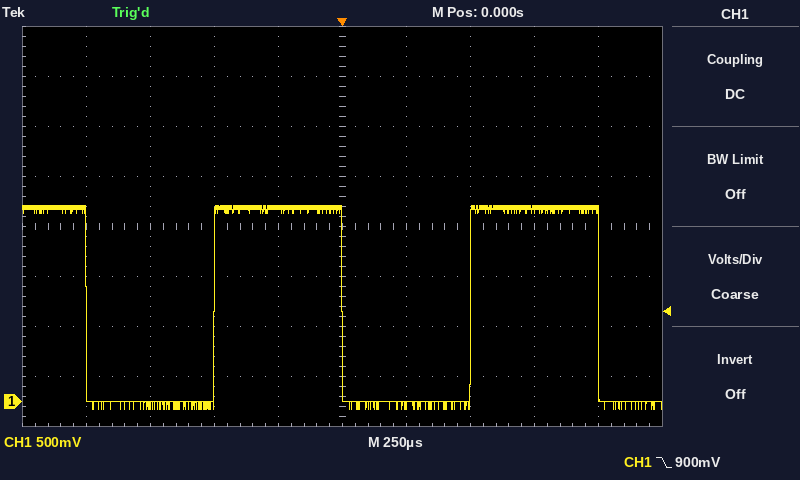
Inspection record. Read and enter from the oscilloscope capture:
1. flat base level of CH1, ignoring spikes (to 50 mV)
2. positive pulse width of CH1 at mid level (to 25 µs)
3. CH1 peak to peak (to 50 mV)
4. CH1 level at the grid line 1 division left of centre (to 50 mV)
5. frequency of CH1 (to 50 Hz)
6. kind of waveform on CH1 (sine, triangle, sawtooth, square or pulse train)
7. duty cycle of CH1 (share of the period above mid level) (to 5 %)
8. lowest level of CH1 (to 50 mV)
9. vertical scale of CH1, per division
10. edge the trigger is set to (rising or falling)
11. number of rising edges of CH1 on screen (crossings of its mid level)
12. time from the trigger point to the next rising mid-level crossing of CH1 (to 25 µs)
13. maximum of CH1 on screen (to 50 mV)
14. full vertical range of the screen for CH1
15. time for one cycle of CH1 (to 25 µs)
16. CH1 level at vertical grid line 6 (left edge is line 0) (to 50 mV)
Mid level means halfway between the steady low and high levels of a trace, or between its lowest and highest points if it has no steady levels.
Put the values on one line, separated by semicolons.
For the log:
0 mV; 500 µs; 2.05 V; 1.95 V; 1.00 kHz; square; 50 %; -100 mV; 500 mV; falling; 2; 500 µs; 1.95 V; 4 V; 1.000 ms; -50 mV
